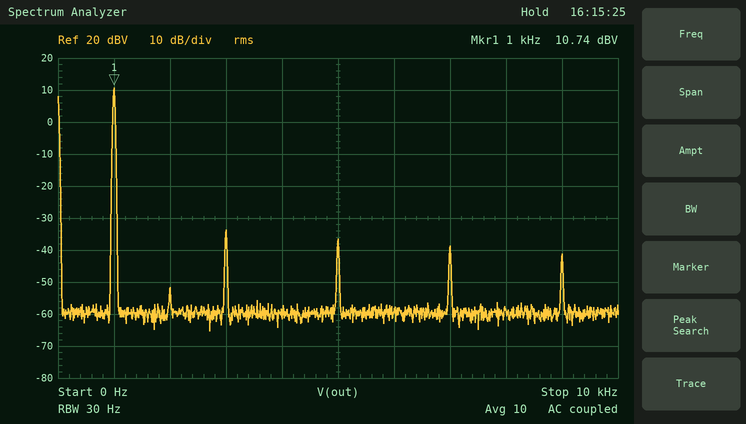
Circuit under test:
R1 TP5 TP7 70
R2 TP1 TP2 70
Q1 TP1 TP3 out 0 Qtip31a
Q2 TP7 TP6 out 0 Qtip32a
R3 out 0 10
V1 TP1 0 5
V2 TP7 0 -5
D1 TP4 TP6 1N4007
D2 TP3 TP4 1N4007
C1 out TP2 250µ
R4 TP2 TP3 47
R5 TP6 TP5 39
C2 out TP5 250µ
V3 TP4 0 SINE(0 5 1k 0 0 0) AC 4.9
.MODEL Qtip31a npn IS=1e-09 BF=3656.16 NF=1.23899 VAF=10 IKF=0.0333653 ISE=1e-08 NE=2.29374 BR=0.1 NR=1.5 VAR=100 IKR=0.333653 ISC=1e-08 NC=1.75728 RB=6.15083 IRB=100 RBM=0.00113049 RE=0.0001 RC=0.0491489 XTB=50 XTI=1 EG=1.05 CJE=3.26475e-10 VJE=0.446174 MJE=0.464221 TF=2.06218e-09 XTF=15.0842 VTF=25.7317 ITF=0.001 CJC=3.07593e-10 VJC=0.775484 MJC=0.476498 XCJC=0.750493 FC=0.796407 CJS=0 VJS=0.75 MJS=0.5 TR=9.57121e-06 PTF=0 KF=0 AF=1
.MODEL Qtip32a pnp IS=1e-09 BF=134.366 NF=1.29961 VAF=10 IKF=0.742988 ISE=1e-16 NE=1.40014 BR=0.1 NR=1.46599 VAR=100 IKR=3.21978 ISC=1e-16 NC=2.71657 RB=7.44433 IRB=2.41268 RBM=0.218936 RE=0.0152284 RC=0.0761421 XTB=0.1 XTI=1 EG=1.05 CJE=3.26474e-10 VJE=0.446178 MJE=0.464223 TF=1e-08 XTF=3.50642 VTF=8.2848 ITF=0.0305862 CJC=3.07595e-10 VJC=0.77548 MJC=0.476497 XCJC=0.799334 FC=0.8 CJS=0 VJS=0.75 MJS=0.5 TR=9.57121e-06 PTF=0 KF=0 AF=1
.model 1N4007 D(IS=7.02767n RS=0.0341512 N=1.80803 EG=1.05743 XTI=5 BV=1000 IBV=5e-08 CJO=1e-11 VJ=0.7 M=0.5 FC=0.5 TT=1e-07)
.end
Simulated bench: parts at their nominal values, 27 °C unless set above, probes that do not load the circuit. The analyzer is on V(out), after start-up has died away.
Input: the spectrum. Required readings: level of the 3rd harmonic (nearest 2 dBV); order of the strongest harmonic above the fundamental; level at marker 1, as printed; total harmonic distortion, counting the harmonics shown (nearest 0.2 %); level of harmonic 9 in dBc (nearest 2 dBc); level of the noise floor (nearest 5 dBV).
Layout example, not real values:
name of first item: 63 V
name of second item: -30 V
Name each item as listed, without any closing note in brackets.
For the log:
level of the 3rd harmonic: -34 dBV
order of the strongest harmonic above the fundamental: 3
level at marker 1, as printed: 10.74 dBV
total harmonic distortion, counting the harmonics shown: 0.8 %
level of harmonic 9 in dBc: -52 dBc
level of the noise floor: -60 dBV
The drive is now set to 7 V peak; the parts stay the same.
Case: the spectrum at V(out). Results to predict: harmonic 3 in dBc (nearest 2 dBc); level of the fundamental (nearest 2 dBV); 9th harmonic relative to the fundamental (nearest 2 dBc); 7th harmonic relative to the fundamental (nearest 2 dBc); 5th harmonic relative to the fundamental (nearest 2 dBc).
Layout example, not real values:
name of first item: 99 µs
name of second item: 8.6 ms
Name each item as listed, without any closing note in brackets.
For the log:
harmonic 3 in dBc: -18 dBc
level of the fundamental: 12 dBV
9th harmonic relative to the fundamental: -42 dBc
7th harmonic relative to the fundamental: -34 dBc
5th harmonic relative to the fundamental: -32 dBc
